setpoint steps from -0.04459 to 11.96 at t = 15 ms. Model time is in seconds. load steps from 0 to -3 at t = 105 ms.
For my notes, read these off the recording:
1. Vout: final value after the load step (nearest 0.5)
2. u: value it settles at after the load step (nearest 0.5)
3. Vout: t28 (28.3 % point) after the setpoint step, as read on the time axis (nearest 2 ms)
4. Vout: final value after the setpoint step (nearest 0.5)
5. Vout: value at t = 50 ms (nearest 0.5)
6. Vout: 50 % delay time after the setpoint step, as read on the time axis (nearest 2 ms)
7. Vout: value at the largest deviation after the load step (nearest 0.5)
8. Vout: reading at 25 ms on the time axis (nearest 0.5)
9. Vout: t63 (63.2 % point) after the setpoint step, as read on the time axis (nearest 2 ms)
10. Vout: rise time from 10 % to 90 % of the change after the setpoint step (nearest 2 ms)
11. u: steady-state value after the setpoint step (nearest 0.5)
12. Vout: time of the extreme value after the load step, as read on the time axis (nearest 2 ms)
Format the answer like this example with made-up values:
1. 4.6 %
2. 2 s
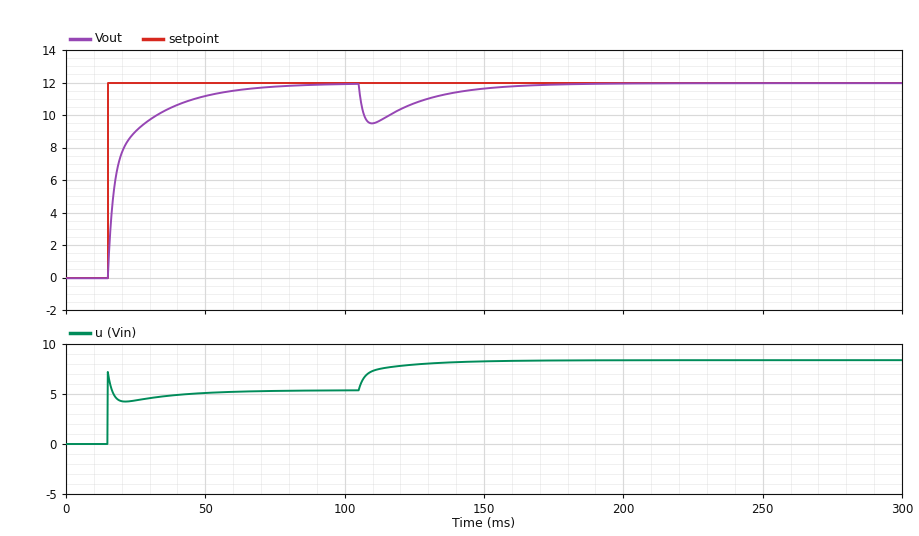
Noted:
1. 12.0
2. 8.5
3. 16 ms
4. 12.0
5. 11.0
6. 18 ms
7. 9.5
8. 9.0
9. 20 ms
10. 26 ms
11. 5.5
12. 110 ms
